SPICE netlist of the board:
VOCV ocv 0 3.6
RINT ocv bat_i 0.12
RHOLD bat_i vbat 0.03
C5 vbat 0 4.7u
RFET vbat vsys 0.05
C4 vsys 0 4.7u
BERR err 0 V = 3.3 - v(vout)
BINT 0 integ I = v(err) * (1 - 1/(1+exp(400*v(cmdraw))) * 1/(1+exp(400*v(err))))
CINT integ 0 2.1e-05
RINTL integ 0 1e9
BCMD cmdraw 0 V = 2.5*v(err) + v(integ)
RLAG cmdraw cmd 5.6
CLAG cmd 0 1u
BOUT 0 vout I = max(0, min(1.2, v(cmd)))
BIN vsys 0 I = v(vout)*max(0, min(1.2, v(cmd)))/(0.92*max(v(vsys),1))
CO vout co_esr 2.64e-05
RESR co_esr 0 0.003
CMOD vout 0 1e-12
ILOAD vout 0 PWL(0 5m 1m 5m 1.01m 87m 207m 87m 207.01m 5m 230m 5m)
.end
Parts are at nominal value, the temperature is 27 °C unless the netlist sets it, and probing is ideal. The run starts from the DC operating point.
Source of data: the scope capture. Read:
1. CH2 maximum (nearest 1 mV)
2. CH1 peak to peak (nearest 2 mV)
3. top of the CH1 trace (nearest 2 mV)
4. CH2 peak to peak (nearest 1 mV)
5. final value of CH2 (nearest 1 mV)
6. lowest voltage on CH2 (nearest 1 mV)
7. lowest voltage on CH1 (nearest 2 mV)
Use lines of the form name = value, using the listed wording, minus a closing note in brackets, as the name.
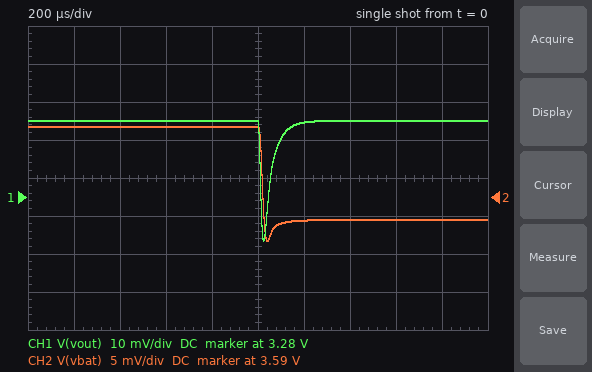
CH2 maximum = 3.599 V
CH1 peak to peak = 32 mV
top of the CH1 trace = 3.300 V
CH2 peak to peak = 15 mV
final value of CH2 = 3.587 V
lowest voltage on CH2 = 3.584 V
lowest voltage on CH1 = 3.268 V
